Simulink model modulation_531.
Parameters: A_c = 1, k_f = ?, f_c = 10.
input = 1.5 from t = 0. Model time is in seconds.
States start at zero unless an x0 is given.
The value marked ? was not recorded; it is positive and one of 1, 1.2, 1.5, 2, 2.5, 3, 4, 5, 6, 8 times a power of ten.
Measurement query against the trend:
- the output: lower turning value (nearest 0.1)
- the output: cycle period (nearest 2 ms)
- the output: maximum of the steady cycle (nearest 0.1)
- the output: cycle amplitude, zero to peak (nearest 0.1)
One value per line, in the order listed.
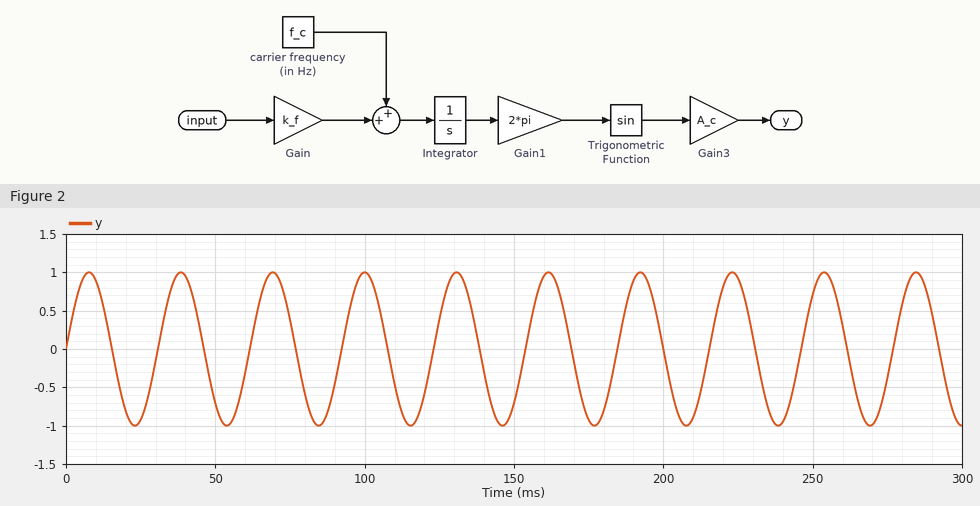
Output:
-1.0
30 ms
1.0
1.0
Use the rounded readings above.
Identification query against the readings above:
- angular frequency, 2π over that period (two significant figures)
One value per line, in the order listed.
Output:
0.21 rad/ms
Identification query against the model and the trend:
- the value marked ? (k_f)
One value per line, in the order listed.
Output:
15
